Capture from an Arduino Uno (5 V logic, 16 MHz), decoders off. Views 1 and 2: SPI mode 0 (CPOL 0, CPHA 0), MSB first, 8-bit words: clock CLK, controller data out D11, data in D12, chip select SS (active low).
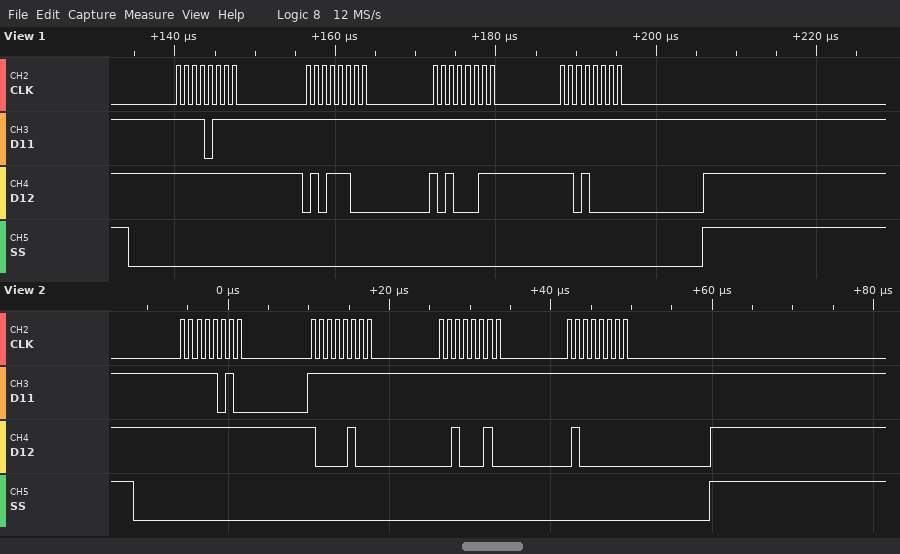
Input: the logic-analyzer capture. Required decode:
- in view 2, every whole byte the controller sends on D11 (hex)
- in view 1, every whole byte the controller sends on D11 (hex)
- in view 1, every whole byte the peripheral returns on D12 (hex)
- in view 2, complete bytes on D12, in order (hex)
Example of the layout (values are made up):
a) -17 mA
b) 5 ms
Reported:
a) 0xFA 0xFF 0xFF 0xFF
b) F7 FF FF FF
c) FF 5C A3 D0
d) 0xFF 0x84 0x22 0x40
